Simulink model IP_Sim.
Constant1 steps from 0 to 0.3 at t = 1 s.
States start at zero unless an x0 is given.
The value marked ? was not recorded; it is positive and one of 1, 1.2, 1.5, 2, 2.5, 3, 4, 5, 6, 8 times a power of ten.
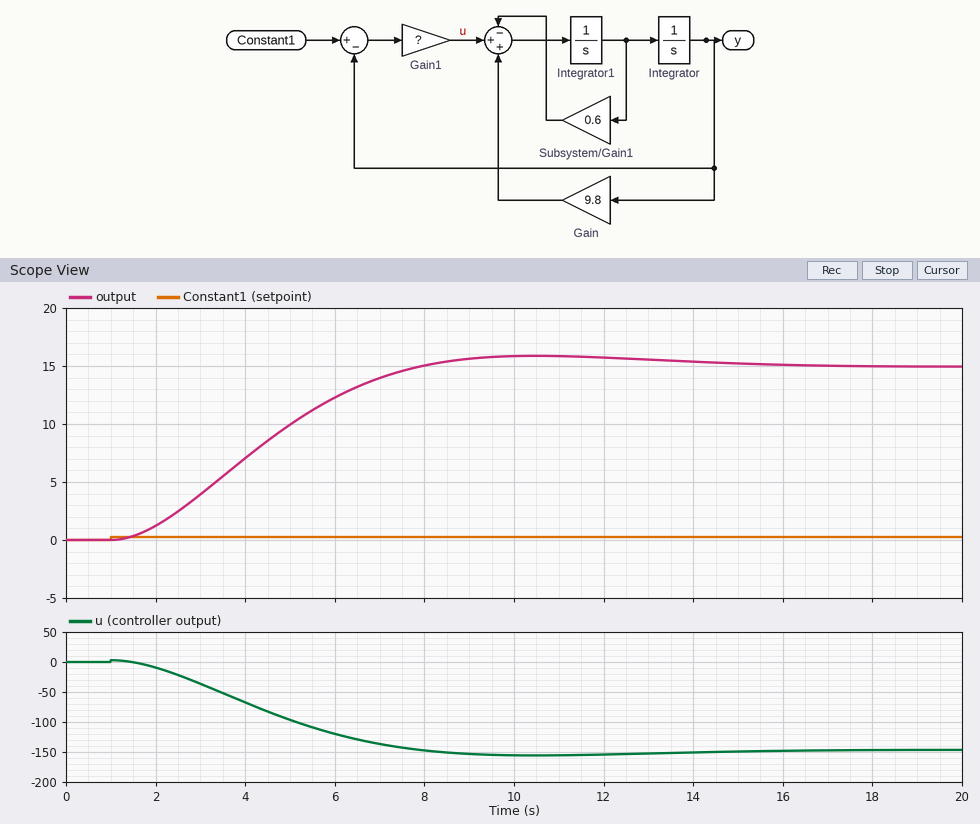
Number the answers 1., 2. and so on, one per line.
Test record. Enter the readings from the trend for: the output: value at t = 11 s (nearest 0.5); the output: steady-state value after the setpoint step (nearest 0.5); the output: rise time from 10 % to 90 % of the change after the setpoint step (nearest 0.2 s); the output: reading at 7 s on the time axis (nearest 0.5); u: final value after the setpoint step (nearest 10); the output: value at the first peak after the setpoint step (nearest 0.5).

1. 16.0
2. 15.0
3. 4.6 s
4. 14.0
5. -150
6. 16.0
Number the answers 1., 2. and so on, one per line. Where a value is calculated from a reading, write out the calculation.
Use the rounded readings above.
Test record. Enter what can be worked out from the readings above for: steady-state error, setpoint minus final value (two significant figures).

1. 0.3 - 15 = -15
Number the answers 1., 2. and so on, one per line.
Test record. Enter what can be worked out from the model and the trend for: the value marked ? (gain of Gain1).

1. 10
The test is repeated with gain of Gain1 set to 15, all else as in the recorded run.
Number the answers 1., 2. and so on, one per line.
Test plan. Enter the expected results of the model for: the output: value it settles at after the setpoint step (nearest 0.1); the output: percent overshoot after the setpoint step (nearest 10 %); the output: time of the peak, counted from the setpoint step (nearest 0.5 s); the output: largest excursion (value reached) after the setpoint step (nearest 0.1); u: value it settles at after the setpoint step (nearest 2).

1. 0.9
2. 70 %
3. 1.5 s
4. 1.4
5. -8
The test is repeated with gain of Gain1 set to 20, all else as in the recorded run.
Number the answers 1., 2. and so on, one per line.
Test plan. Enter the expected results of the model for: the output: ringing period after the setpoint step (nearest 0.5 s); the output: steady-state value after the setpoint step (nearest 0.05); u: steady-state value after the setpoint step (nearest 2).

1. 2.0 s
2. 0.60
3. -6
